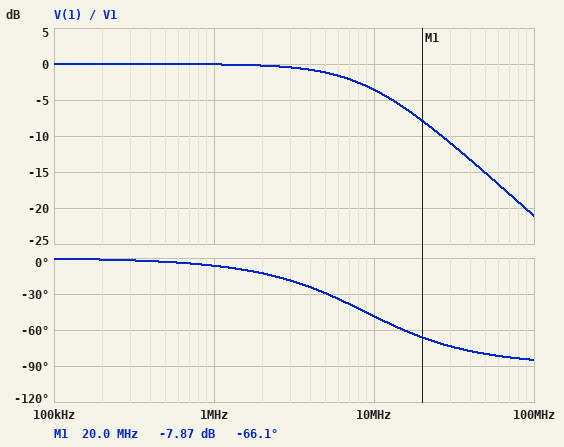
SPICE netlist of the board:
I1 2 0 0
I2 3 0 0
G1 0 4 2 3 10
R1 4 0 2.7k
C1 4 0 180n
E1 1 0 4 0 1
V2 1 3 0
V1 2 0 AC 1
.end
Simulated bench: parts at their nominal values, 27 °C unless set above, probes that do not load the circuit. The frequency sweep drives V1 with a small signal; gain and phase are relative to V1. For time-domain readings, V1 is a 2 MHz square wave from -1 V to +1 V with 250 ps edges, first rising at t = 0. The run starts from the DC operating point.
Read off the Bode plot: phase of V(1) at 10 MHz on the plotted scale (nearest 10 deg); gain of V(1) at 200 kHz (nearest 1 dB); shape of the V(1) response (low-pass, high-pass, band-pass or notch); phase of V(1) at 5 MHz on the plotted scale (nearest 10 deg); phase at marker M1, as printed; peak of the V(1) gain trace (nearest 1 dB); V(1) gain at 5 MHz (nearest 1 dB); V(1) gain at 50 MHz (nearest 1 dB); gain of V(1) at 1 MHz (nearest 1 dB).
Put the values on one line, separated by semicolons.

-50 deg; 0 dB; low-pass; -30 deg; -66.1 deg; 0 dB; -1 dB; -15 dB; 0 dB
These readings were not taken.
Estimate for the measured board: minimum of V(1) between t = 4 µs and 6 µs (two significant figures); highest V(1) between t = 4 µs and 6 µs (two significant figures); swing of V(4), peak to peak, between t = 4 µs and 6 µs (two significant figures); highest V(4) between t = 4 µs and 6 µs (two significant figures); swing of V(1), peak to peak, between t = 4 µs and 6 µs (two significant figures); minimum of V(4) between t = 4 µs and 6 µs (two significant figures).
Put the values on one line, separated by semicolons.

-1.0 V; 1.0 V; 2.0 V; 1.0 V; 2.0 V; -1.0 V
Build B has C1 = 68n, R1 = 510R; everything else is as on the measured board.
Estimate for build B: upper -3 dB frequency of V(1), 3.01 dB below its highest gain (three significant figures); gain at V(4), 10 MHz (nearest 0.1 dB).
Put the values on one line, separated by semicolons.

23.4 MHz; -0.7 dB
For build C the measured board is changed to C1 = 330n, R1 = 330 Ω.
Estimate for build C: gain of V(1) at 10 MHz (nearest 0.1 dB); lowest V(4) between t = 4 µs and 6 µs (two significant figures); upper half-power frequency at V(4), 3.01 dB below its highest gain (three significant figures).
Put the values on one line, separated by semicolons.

-7.2 dB; -1.0 V; 4.82 MHz
